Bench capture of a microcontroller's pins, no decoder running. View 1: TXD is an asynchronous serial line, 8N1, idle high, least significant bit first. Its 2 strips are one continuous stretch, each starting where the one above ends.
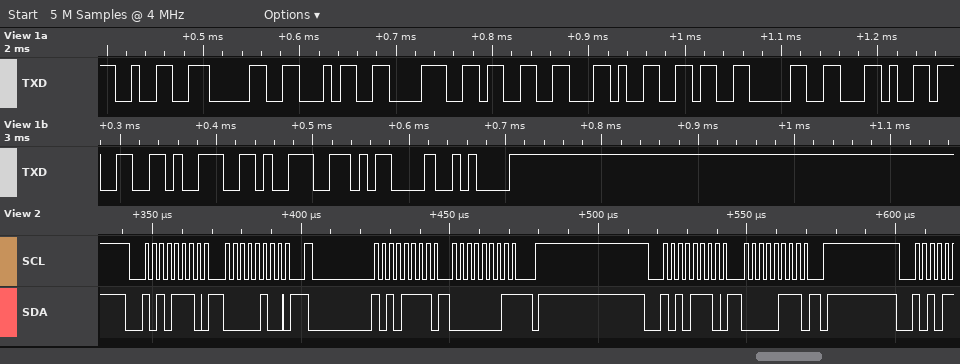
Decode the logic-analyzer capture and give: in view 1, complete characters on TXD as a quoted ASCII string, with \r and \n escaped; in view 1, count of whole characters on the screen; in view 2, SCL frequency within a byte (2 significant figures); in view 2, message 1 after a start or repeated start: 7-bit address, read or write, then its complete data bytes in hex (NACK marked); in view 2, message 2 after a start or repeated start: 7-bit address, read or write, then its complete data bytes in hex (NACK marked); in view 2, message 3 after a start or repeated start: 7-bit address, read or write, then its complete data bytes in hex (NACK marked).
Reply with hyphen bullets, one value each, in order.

- "20483,60,399\r\n"
- 14
- 400 kHz
- 0x57 write: 04
- 0x57 read: 01 NACK
- 0x57 write: 07
